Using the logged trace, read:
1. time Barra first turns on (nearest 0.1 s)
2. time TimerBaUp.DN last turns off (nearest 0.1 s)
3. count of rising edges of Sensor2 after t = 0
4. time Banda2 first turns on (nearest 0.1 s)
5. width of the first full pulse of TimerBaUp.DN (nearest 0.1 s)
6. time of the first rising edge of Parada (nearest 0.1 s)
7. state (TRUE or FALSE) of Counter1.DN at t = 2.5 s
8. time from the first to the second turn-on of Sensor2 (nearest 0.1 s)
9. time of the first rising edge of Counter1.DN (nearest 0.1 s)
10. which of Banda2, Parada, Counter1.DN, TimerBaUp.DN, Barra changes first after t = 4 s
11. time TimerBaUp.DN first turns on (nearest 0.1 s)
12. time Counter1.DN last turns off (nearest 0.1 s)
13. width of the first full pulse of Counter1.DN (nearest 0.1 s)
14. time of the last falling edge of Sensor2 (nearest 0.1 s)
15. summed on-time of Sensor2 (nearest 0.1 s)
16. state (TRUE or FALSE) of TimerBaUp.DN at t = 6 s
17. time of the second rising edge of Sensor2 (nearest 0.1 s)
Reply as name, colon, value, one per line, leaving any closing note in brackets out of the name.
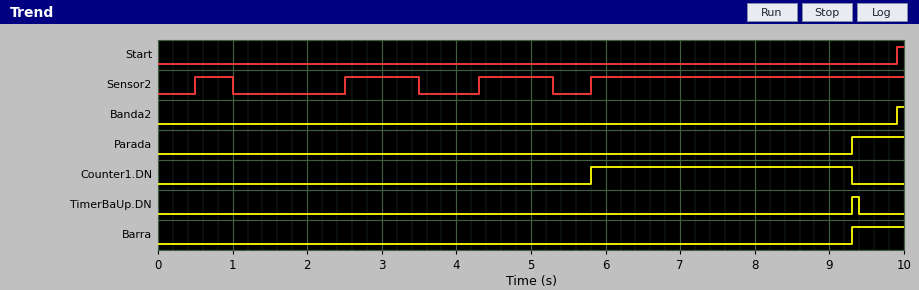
time Barra first turns on: 9.3 s
time TimerBaUp.DN last turns off: 9.4 s
count of rising edges of Sensor2 after t = 0: 4
time Banda2 first turns on: 9.9 s
width of the first full pulse of TimerBaUp.DN: 0.1 s
time of the first rising edge of Parada: 9.3 s
state (TRUE or FALSE) of Counter1.DN at t = 2.5 s: FALSE
time from the first to the second turn-on of Sensor2: 2.0 s
time of the first rising edge of Counter1.DN: 5.8 s
which of Banda2, Parada, Counter1.DN, TimerBaUp.DN, Barra changes first after t = 4 s: Counter1.DN
time TimerBaUp.DN first turns on: 9.3 s
time Counter1.DN last turns off: 9.3 s
width of the first full pulse of Counter1.DN: 3.5 s
time of the last falling edge of Sensor2: 5.3 s
summed on-time of Sensor2: 6.7 s
state (TRUE or FALSE) of TimerBaUp.DN at t = 6 s: FALSE
time of the second rising edge of Sensor2: 2.5 s
